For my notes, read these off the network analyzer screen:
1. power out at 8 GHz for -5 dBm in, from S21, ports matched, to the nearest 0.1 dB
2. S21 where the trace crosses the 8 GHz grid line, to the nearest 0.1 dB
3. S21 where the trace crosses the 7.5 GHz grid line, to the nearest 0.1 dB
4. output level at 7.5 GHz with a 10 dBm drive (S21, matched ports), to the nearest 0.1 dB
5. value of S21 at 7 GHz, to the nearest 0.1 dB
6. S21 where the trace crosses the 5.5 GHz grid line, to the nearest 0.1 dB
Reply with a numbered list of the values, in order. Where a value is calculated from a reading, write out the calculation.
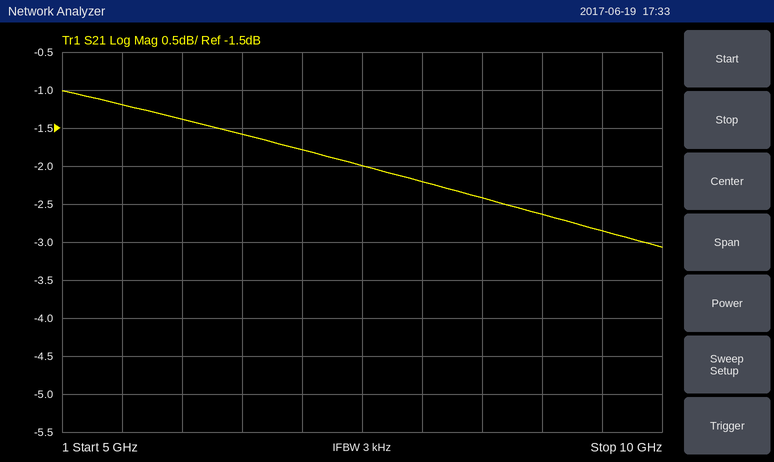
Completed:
1. -5 dBm + (-2.2 dB) = -7.2 dBm
2. -2.2 dB
3. -2.0 dB
4. 10 dBm + (-2.0 dB) = 8.0 dBm
5. -1.8 dB
6. -1.2 dB
